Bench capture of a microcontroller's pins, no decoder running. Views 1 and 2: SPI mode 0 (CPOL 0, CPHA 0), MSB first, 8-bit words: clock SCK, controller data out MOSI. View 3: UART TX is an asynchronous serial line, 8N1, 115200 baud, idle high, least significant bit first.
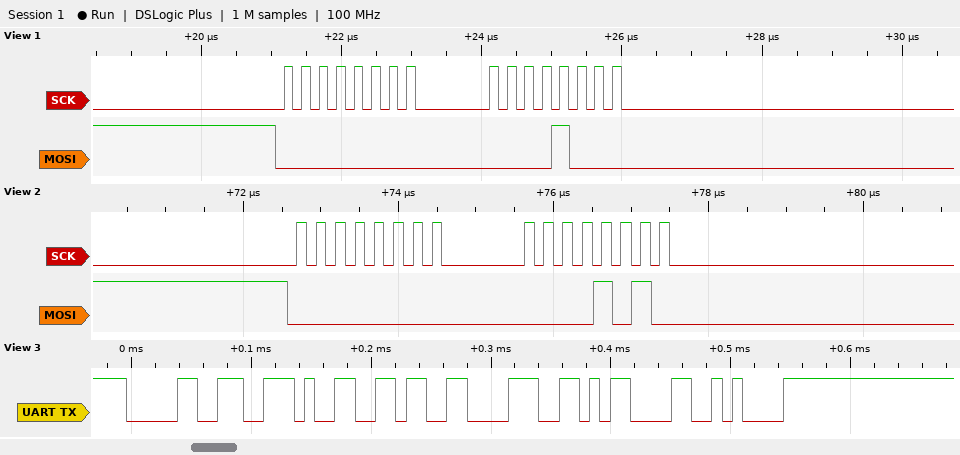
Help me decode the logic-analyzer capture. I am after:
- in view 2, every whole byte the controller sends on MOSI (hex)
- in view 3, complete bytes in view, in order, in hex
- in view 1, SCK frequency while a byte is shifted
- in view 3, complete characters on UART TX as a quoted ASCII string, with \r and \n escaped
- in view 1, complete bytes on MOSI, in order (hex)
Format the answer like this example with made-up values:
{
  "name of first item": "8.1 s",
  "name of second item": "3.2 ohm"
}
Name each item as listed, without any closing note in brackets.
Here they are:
{
  "in view 2, every whole byte the controller sends on MOSI": "00 0A",
  "in view 3, complete bytes in view, in order, in hex": "30 2E 36 38 0D 0A",
  "in view 1, SCK frequency while a byte is shifted": "4 MHz",
  "in view 3, complete characters on UART TX as a quoted ASCII string, with \\r and \\n escaped": "\"0.68\\r\\n\"",
  "in view 1, complete bytes on MOSI, in order": "0x00 0x08"
}
